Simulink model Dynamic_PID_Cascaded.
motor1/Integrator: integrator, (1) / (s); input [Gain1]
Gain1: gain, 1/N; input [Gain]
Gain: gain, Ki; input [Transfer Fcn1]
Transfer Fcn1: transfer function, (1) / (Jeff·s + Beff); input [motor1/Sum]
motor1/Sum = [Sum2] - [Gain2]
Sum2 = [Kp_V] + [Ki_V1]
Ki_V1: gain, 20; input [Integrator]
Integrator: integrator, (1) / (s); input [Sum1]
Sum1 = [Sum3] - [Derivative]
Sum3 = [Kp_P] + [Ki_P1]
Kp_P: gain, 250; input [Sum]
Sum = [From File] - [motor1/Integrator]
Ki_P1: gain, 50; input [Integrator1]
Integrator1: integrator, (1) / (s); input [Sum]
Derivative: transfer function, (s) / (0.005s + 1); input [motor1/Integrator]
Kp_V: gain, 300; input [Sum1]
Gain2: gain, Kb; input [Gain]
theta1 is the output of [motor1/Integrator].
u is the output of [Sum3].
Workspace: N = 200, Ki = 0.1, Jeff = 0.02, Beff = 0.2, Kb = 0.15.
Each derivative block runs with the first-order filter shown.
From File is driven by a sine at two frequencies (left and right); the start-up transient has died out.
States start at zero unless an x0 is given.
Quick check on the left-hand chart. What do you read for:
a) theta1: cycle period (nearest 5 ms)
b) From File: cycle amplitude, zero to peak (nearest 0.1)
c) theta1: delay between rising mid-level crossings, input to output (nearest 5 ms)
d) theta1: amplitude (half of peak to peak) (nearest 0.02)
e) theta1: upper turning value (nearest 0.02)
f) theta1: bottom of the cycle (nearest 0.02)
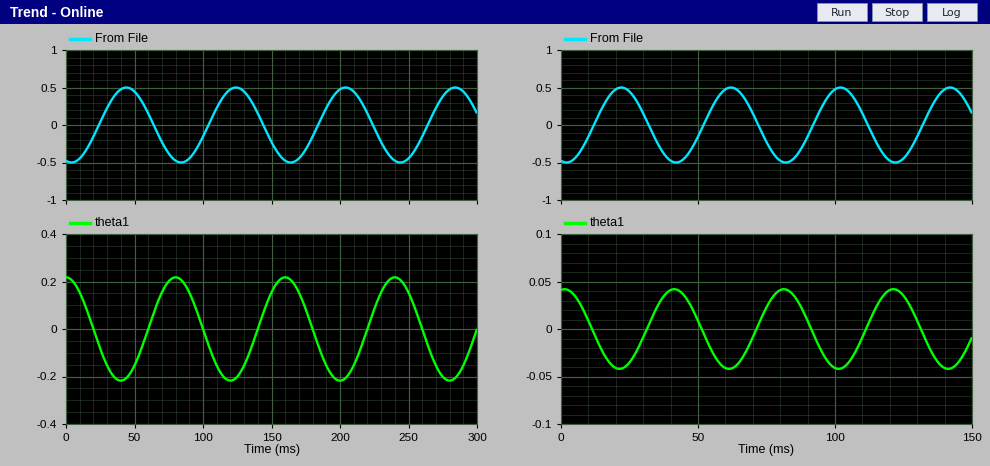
80 ms
0.5
35 ms
0.22
0.22
-0.22
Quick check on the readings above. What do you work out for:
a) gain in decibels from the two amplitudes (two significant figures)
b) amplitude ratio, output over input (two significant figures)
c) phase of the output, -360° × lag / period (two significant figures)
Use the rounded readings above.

-7.1 dB
0.44
-160°
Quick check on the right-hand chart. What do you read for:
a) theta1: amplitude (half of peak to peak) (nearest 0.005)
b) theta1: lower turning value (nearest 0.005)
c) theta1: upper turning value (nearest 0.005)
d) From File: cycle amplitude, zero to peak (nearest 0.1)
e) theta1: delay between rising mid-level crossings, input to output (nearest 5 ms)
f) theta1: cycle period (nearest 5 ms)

0.040
-0.040
0.040
0.5
20 ms
40 ms
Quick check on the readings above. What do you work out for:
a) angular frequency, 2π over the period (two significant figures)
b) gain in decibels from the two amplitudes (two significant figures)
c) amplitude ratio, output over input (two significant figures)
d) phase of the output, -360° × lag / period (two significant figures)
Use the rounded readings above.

0.16 rad/ms
-22 dB
0.080
-180°
